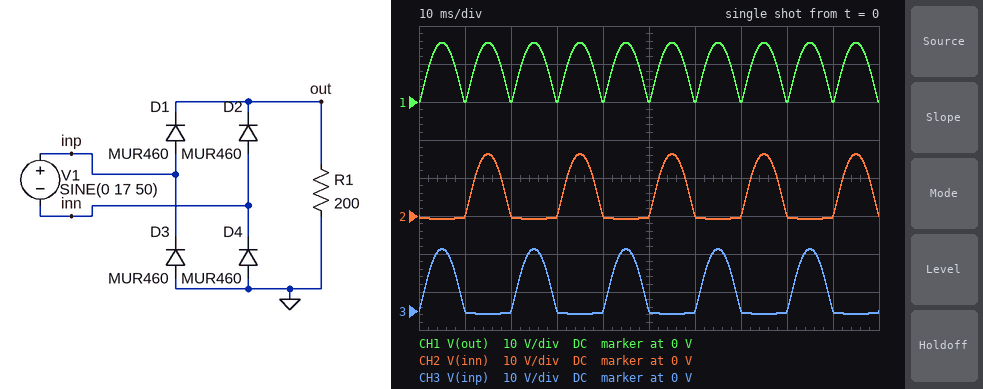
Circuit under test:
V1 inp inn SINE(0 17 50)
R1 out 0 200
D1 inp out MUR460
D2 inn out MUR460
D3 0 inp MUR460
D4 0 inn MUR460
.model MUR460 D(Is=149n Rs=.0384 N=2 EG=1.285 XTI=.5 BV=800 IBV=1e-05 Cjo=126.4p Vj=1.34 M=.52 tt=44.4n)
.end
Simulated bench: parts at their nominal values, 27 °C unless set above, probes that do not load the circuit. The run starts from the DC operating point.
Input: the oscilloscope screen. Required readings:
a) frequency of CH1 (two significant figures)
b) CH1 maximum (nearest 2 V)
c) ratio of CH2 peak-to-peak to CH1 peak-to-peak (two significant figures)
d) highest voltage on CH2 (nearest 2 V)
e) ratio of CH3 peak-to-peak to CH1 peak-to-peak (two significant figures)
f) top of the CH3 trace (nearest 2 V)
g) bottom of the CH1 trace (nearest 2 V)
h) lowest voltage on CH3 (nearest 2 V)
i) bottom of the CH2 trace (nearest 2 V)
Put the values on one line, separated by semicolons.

100 Hz; 16 V; 1.1; 16 V; 1.1; 16 V; 0 V; 0 V; 0 V
